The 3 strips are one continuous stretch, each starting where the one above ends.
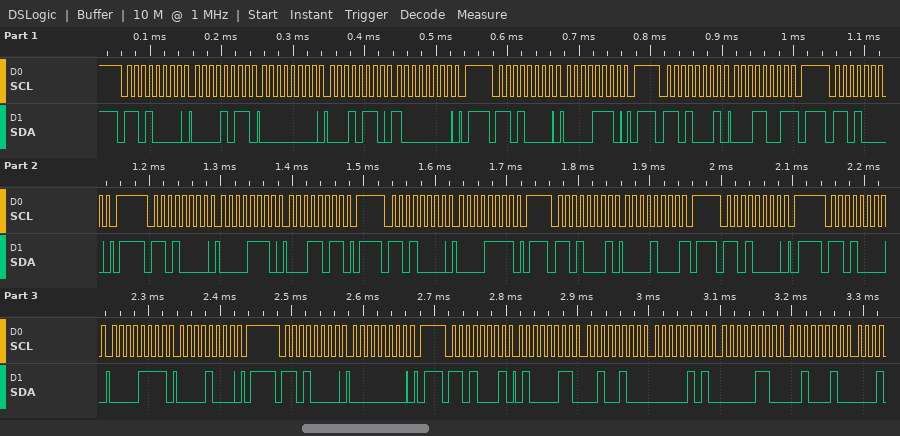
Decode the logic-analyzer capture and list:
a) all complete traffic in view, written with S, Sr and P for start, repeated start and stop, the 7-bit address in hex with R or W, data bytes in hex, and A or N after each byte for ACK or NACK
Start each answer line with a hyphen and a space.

- S 68W A 0B A 00 A 16 A 80 A P S 68W A 0E A P S 68R A 19 N P S 68W A P S 68W A 0E A 1B A P S 68W A 0F A P S 68R A 08 N P S 68W A P S 68W A 0F A 08 A P S 68W A 00 A P S 68R A 43 A 24 A 05 A 06 A 22 A
